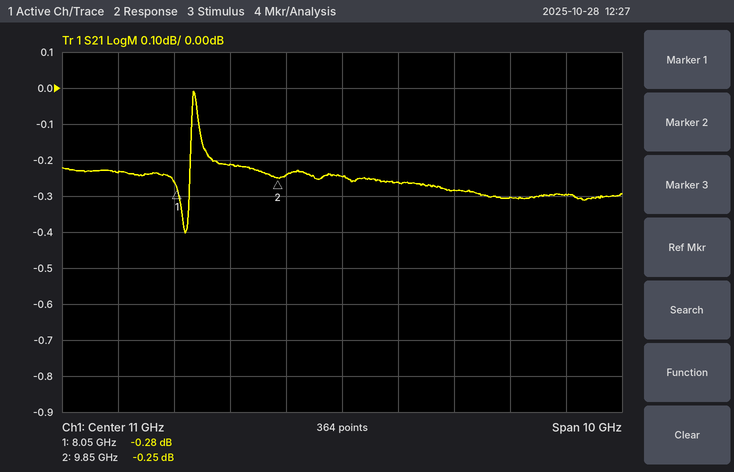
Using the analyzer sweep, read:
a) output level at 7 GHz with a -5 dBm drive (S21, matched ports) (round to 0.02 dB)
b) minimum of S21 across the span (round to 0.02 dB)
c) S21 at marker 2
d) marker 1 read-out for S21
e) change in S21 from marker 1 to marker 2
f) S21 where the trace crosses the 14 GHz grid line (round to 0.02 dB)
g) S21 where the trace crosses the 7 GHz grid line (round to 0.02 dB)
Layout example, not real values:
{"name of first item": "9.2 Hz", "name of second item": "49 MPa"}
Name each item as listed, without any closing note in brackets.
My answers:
{"output level at 7 GHz with a -5 dBm drive (S21, matched ports)": "-5.24 dBm", "minimum of S21 across the span": "-0.40 dB", "S21 at marker 2": "-0.25 dB", "marker 1 read-out for S21": "-0.28 dB", "change in S21 from marker 1 to marker 2": "0.03 dB", "S21 where the trace crosses the 14 GHz grid line": "-0.30 dB", "S21 where the trace crosses the 7 GHz grid line": "-0.24 dB"}
